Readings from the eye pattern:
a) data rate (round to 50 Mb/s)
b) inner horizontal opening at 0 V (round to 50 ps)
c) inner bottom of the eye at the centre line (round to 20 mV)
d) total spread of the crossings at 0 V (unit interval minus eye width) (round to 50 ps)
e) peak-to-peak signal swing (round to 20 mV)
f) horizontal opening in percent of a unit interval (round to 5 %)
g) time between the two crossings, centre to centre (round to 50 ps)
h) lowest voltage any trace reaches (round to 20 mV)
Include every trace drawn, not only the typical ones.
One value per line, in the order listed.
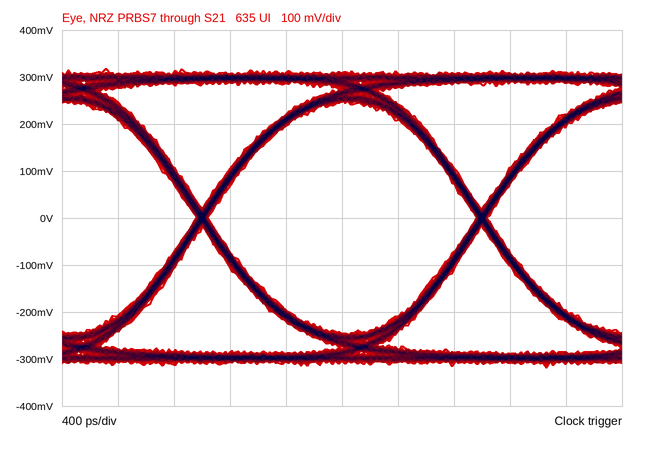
500 Mb/s
1.90 ns
-240 mV
100 ps
640 mV
95 %
2.00 ns
-320 mV
